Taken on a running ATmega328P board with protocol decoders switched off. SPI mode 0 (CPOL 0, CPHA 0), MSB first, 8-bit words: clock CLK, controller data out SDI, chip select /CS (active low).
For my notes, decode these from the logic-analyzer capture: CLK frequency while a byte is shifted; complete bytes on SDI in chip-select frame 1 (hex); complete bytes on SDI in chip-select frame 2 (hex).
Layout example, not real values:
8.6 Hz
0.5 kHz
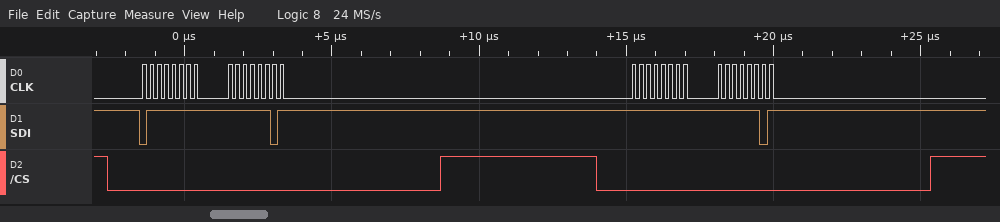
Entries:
4 MHz
7F FD
FF FD
